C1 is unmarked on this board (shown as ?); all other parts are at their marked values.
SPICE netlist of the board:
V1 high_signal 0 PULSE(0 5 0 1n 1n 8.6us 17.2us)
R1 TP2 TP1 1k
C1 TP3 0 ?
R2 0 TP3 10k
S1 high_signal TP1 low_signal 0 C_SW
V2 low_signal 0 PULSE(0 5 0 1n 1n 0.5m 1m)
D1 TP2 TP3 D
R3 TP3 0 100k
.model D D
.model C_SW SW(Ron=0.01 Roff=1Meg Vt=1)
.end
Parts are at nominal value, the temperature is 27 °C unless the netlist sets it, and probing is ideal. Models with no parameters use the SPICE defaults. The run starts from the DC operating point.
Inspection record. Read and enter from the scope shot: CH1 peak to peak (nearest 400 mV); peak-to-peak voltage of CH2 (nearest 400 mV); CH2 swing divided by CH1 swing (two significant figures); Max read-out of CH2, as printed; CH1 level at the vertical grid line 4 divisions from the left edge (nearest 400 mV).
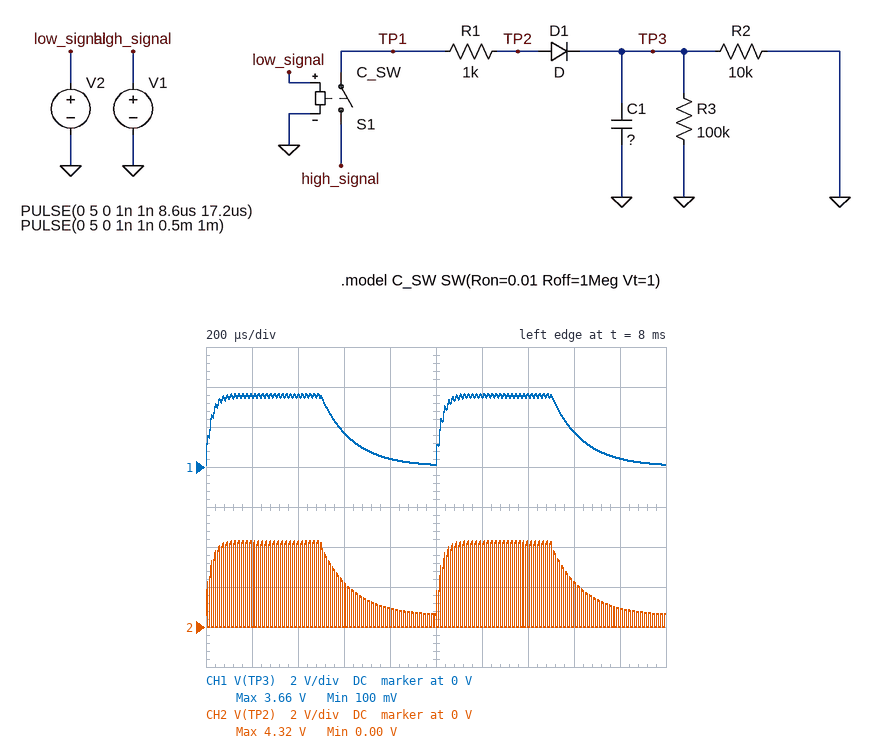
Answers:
3.6 V
4.4 V
1.2
4.32 V
400 mV
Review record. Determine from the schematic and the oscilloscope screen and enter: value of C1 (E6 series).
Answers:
15 nF
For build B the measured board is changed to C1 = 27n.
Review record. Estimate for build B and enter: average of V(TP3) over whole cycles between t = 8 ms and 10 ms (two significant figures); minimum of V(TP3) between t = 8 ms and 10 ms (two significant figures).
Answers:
2.4 V
470 mV
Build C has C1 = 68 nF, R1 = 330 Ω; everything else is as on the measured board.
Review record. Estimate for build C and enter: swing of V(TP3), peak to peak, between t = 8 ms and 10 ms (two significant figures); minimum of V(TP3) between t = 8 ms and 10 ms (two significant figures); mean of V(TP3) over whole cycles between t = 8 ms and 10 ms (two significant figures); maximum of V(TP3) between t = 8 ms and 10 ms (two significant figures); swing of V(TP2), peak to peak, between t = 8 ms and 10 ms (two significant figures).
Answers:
2.3 V
1.8 V
3.3 V
4.1 V
4.7 V
